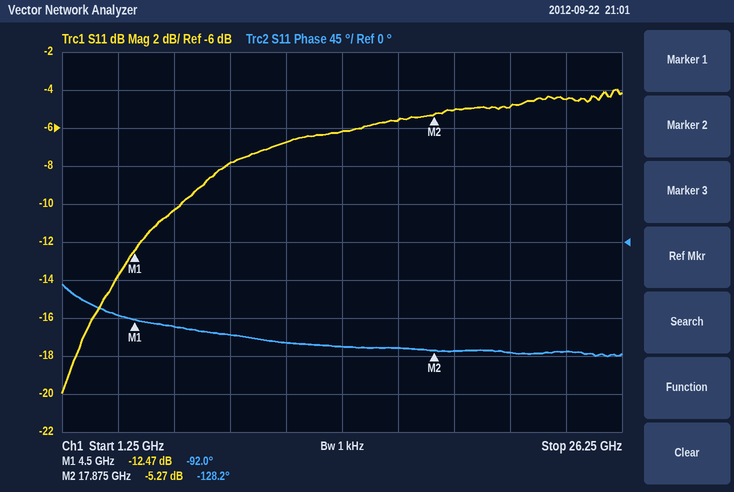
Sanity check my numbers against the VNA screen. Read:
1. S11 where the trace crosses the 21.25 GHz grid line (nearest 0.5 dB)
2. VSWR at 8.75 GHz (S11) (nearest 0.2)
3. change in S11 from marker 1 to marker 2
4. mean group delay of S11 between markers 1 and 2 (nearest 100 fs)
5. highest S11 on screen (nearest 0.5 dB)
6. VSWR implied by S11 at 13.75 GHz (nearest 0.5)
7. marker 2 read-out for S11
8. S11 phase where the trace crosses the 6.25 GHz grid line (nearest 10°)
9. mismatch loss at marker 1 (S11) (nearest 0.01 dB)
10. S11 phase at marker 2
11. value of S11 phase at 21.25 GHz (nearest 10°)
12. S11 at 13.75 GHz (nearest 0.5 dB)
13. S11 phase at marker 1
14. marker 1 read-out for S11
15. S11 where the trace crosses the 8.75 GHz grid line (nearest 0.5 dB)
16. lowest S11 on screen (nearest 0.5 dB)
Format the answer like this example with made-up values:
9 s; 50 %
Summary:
-5.0 dB; 2.4; 7.20 dB; 7.5 ps; -4.0 dB; 3.0; -5.27 dB; -100°; 0.25 dB; -128.2°; -130°; -6.0 dB; -92.0°; -12.47 dB; -8.0 dB; -20.0 dB
